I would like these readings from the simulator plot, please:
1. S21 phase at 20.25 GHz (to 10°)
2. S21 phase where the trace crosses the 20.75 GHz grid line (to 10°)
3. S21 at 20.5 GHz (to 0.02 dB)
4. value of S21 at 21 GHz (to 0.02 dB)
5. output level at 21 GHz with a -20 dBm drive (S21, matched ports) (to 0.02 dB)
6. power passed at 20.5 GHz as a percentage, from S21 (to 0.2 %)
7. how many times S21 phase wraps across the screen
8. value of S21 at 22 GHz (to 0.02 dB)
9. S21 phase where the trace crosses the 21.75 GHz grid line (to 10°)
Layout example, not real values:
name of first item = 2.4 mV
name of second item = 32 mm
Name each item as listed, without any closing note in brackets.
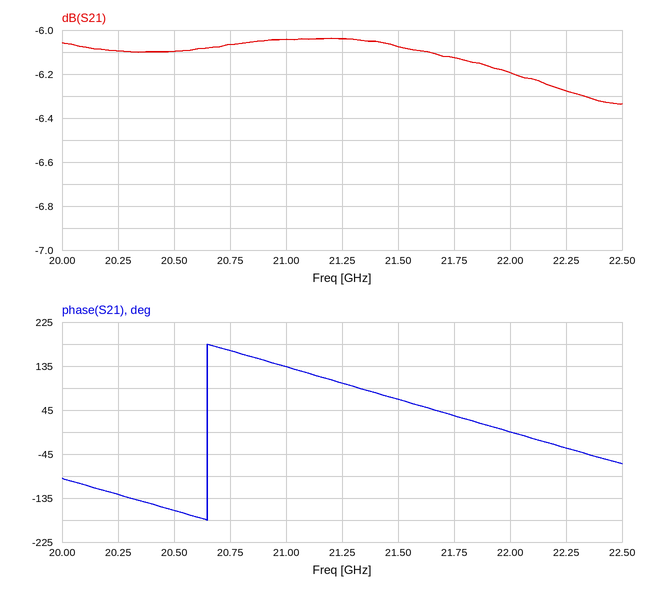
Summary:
S21 phase at 20.25 GHz = -130°
S21 phase where the trace crosses the 20.75 GHz grid line = 170°
S21 at 20.5 GHz = -6.10 dB
value of S21 at 21 GHz = -6.04 dB
output level at 21 GHz with a -20 dBm drive (S21, matched ports) = -26.04 dBm
power passed at 20.5 GHz as a percentage, from S21 = 24.6 %
how many times S21 phase wraps across the screen = 1
value of S21 at 22 GHz = -6.20 dB
S21 phase where the trace crosses the 21.75 GHz grid line = 30°
